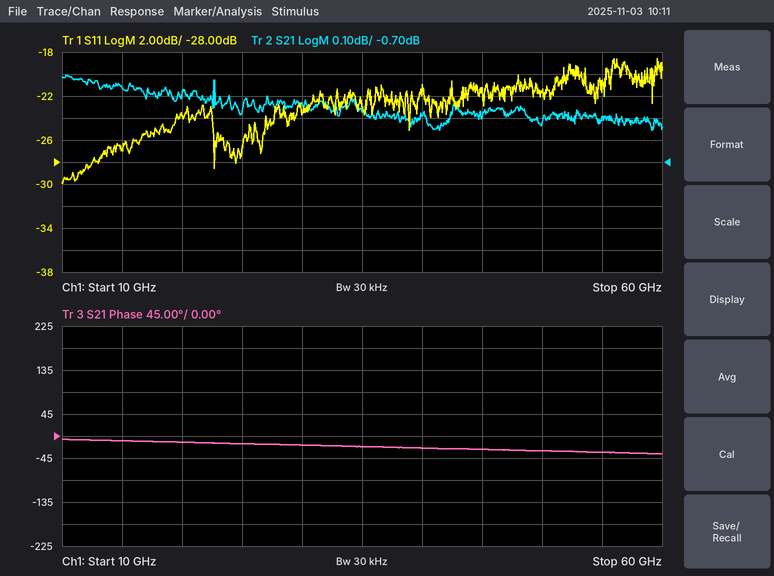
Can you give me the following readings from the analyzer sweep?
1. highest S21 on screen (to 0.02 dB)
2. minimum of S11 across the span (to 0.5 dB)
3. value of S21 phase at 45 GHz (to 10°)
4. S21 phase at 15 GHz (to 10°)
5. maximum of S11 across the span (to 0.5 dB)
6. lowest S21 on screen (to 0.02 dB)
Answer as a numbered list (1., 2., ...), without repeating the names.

1. -0.30 dB
2. -30.0 dB
3. -30°
4. -10°
5. -18.5 dB
6. -0.56 dB
